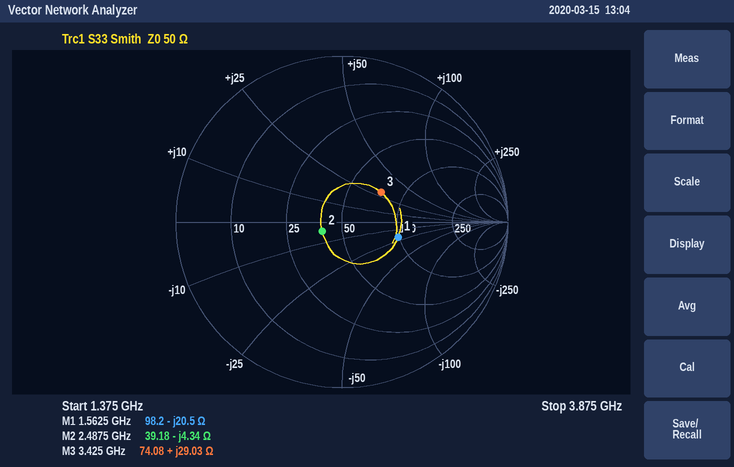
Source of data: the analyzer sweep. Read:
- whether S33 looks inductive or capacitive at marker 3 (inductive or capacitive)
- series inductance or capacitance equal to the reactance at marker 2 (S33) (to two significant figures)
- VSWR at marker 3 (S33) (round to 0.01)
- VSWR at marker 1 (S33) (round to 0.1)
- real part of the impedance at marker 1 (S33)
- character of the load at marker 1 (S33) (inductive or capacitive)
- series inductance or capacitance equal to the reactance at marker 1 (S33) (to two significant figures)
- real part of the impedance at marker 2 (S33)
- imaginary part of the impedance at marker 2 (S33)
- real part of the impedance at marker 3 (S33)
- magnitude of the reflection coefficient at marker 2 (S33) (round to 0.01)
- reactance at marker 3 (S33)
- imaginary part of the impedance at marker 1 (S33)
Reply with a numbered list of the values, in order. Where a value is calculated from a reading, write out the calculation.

1. inductive
2. C = 1/(2π × 2.4875 GHz × 4.34 Ω) ≈ 15 pF
3. 1.84
4. 2.1
5. 98.2 Ω
6. capacitive
7. C = 1/(2π × 1.5625 GHz × 20.5 Ω) ≈ 5.0 pF
8. 39.18 Ω
9. -4.34 Ω
10. 74.08 Ω
11. 0.13
12. +29.03 Ω
13. -20.5 Ω
